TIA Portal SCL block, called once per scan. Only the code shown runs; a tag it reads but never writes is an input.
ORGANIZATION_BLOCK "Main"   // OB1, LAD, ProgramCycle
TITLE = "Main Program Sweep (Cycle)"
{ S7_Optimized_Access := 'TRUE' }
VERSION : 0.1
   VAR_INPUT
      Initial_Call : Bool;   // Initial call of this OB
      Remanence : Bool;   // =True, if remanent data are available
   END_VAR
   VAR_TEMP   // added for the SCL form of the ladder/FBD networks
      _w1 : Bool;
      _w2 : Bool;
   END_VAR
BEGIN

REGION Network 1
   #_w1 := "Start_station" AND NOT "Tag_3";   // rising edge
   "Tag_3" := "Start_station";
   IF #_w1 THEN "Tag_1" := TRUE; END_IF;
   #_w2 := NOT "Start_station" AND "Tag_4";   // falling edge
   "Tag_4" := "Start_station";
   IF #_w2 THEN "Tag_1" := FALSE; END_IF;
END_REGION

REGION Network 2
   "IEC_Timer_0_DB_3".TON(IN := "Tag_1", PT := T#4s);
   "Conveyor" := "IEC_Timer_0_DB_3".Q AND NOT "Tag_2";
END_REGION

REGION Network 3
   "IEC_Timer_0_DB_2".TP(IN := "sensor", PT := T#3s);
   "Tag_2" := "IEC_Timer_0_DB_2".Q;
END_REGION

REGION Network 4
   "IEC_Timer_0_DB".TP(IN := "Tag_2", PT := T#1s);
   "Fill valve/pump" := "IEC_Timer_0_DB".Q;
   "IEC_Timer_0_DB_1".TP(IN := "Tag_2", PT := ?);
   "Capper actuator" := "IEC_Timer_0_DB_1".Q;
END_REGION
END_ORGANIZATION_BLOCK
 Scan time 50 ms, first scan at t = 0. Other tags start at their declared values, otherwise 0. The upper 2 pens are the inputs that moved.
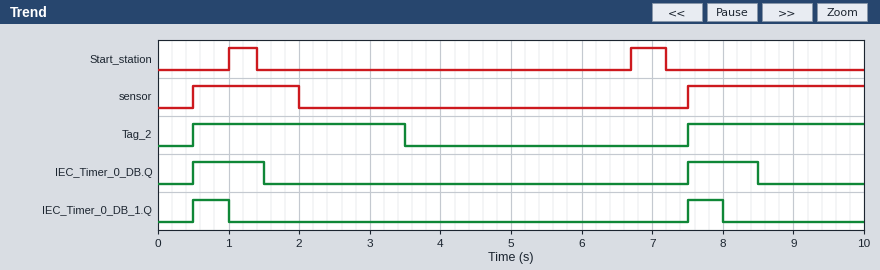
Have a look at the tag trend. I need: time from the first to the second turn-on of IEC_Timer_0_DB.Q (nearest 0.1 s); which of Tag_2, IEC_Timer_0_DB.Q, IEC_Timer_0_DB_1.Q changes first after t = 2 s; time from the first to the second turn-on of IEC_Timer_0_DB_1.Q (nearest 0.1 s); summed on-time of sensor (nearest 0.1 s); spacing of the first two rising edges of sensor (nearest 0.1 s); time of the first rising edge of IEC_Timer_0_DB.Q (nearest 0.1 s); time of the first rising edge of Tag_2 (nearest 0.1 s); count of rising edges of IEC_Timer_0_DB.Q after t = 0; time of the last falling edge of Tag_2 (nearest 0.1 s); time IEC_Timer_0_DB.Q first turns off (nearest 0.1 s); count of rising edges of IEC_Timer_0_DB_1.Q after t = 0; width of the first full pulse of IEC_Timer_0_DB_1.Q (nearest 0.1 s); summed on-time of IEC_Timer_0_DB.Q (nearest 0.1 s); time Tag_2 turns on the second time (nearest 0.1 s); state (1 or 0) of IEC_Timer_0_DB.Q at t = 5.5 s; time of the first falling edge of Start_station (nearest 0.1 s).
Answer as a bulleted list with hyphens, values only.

- 7.0 s
- Tag_2
- 7.0 s
- 4.0 s
- 7.0 s
- 0.5 s
- 0.5 s
- 2
- 3.5 s
- 1.5 s
- 2
- 0.5 s
- 2.0 s
- 7.5 s
- 0
- 1.4 s
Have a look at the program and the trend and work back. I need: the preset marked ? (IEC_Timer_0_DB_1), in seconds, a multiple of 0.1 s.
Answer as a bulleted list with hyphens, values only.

- 0.5 s
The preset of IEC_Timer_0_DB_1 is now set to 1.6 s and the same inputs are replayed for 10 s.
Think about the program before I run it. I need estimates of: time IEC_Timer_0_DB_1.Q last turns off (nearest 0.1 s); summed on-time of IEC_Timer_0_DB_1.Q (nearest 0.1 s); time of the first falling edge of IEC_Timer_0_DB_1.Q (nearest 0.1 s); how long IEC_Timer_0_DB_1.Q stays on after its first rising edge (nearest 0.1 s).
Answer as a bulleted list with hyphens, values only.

- 9.1 s
- 3.2 s
- 2.1 s
- 1.6 s
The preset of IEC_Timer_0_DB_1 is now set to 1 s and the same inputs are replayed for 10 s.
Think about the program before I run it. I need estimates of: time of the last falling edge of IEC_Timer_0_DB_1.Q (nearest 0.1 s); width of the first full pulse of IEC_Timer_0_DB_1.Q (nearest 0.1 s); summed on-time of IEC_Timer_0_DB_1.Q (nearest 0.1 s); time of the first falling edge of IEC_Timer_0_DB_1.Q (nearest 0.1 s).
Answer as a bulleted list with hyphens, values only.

- 8.5 s
- 1.0 s
- 2.0 s
- 1.5 s
